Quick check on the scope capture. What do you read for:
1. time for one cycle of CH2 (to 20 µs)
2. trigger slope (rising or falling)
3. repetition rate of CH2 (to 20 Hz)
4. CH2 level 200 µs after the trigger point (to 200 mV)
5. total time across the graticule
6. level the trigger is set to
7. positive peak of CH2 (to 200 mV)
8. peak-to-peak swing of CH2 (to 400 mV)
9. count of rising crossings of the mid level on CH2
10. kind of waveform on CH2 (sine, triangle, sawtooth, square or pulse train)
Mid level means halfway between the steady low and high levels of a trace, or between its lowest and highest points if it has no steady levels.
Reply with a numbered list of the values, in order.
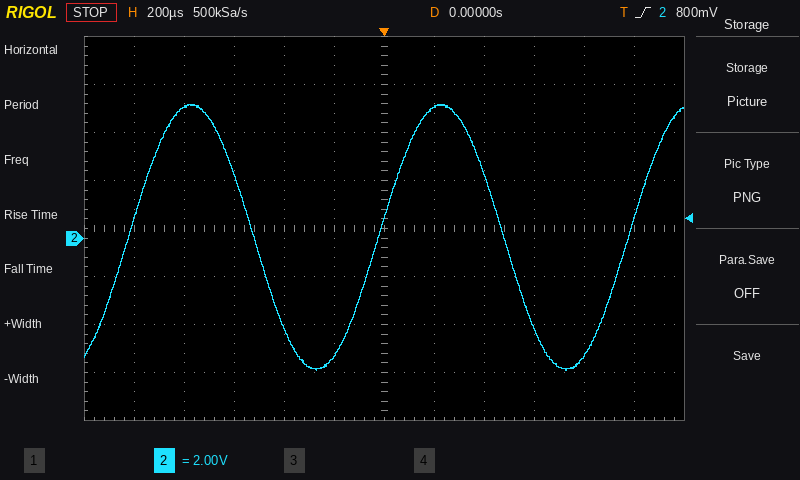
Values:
1. 1.00 ms
2. rising
3. 1.00 kHz
4. 5.4 V
5. 2.4 ms
6. 800 mV
7. 5.6 V
8. 11.2 V
9. 3
10. sine
